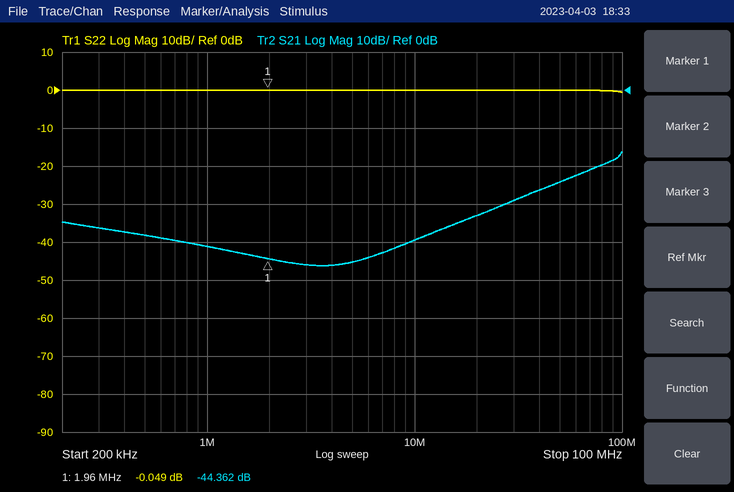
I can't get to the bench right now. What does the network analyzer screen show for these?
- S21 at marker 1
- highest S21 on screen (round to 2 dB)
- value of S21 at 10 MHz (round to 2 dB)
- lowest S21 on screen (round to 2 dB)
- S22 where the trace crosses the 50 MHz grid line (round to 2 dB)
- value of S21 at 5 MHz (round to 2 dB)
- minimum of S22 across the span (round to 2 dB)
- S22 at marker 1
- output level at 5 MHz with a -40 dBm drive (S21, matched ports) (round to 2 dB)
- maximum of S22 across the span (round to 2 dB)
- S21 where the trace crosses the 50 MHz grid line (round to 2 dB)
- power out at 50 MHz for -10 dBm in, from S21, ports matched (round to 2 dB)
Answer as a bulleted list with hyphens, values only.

- -44.362 dB
- -16 dB
- -40 dB
- -46 dB
- 0 dB
- -46 dB
- 0 dB
- -0.049 dB
- -86 dBm
- 0 dB
- -24 dB
- -34 dBm
